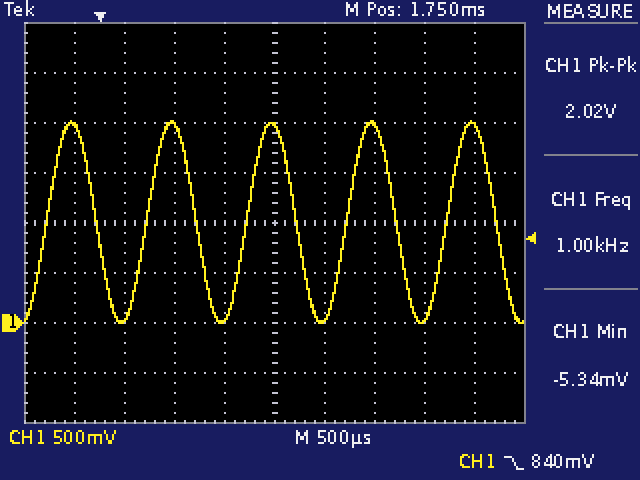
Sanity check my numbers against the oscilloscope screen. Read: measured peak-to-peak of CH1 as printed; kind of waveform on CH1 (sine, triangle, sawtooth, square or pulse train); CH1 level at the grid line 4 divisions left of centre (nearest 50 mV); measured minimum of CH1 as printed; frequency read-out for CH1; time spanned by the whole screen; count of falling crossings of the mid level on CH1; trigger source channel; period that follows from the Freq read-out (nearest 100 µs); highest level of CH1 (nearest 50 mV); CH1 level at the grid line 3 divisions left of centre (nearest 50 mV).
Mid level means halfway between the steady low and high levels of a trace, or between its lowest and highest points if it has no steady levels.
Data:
2.02 V
sine
1.95 V
-5.34 mV
1.00 kHz
5 ms
5
CH1
1.0 ms
2.00 V
50 mV
